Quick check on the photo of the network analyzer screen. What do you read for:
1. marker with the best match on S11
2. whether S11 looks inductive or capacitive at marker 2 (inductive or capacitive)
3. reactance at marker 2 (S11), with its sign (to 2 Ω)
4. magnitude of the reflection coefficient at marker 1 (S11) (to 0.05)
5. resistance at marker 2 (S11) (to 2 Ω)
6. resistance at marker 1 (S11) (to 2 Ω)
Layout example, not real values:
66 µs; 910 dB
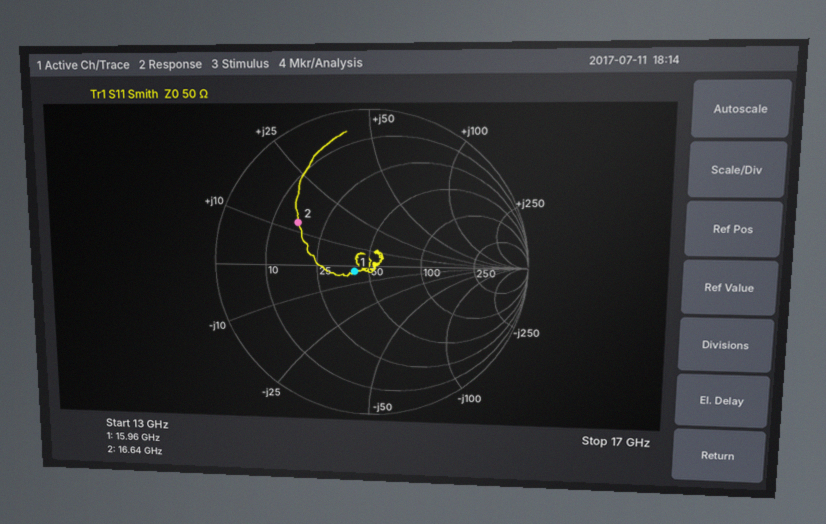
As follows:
marker 1; inductive; +12 Ω; 0.10; 16 Ω; 42 Ω
